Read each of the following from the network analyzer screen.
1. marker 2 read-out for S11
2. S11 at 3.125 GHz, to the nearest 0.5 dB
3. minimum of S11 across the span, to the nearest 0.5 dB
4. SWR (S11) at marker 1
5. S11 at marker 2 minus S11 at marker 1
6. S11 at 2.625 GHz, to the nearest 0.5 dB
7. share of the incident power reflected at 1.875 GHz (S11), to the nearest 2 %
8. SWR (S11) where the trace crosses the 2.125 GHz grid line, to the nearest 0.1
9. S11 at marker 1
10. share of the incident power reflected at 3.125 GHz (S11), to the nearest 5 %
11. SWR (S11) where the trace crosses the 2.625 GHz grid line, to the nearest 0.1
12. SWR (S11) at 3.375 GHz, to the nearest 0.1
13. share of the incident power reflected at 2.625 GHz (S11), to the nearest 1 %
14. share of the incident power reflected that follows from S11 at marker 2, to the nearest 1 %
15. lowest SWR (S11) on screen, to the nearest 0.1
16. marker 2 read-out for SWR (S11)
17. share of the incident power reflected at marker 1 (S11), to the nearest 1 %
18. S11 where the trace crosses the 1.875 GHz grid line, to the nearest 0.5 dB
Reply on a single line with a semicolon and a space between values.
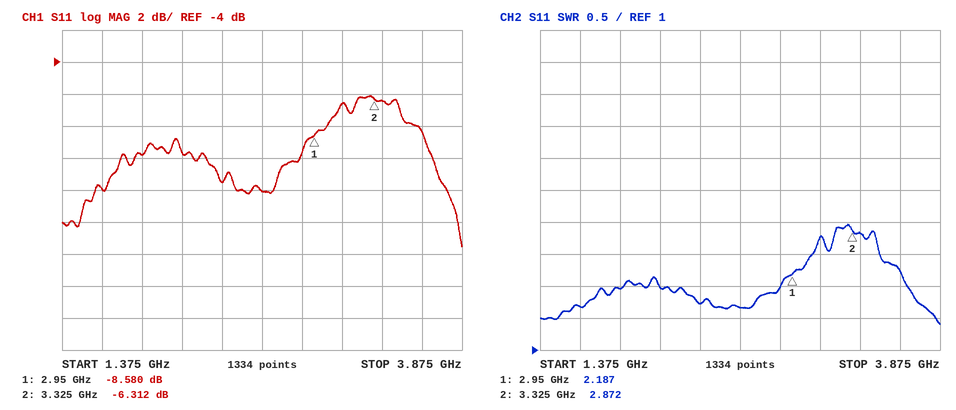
-6.312 dB; -6.5 dB; -15.5 dB; 2.187; 2.268 dB; -12.0 dB; 10 %; 2.0; -8.580 dB; 20 %; 1.7; 2.8; 6 %; 23 %; 1.4; 2.872; 14 %; -10.0 dB
